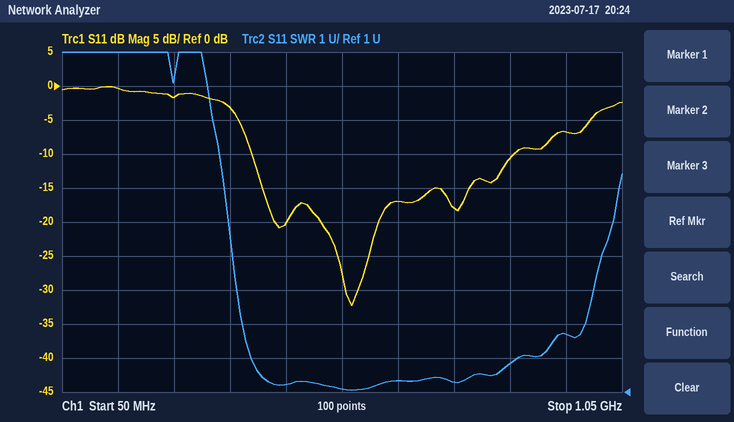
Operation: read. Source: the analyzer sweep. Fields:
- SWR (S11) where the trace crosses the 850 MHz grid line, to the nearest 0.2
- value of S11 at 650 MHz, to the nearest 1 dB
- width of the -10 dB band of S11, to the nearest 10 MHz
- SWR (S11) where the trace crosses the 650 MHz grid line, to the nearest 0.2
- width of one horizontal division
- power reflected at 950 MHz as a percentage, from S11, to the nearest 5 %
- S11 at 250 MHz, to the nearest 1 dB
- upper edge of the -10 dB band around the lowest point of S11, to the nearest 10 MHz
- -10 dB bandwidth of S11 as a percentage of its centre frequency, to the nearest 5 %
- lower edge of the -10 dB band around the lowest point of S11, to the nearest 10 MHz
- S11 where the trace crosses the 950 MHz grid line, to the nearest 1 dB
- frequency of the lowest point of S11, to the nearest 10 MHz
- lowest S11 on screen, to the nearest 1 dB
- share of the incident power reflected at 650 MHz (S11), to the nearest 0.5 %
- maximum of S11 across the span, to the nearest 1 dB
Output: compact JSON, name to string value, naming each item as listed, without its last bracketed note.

{"SWR (S11) where the trace crosses the 850 MHz grid line, to the nearest 0.2": "1.8", "value of S11 at 650 MHz, to the nearest 1 dB": "-17 dB", "width of the -10 dB band of S11, to the nearest 10 MHz": "470 MHz", "SWR (S11) where the trace crosses the 650 MHz grid line, to the nearest 0.2": "1.4", "width of one horizontal division": "100 MHz", "power reflected at 950 MHz as a percentage, from S11, to the nearest 5 %": "20 %", "S11 at 250 MHz, to the nearest 1 dB": "-2 dB", "upper edge of the -10 dB band around the lowest point of S11, to the nearest 10 MHz": "860 MHz", "-10 dB bandwidth of S11 as a percentage of its centre frequency, to the nearest 5 %": "75 %", "lower edge of the -10 dB band around the lowest point of S11, to the nearest 10 MHz": "390 MHz", "S11 where the trace crosses the 950 MHz grid line, to the nearest 1 dB": "-7 dB", "frequency of the lowest point of S11, to the nearest 10 MHz": "570 MHz", "lowest S11 on screen, to the nearest 1 dB": "-32 dB", "share of the incident power reflected at 650 MHz (S11), to the nearest 0.5 %": "2.0 %", "maximum of S11 across the span, to the nearest 1 dB": "0 dB"}
